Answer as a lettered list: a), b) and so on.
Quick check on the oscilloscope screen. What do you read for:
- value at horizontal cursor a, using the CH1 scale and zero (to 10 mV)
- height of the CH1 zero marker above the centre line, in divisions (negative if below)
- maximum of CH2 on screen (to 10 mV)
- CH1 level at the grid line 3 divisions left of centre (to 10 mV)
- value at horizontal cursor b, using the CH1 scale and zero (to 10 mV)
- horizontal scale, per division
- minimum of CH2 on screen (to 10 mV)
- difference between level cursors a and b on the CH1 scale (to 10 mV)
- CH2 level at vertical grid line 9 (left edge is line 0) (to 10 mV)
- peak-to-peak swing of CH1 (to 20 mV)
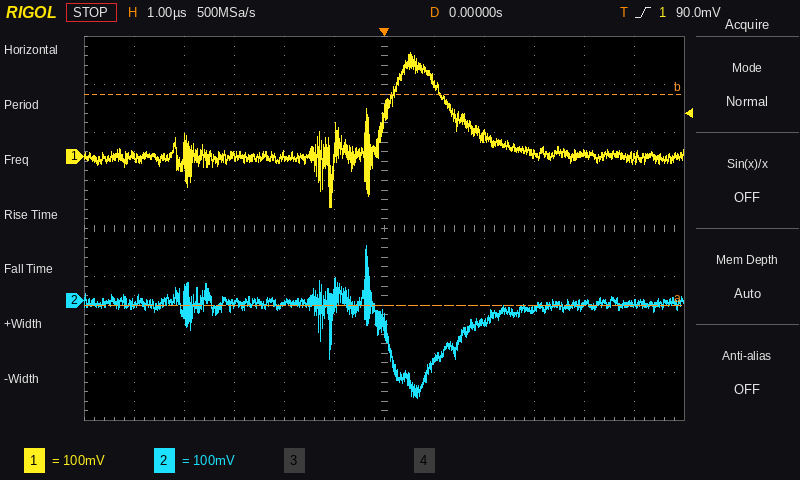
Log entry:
a) -310 mV
b) +1.5 div
c) 110 mV
d) 0 mV
e) 130 mV
f) 1 µs
g) -200 mV
h) 440 mV
i) -20 mV
j) 320 mV
